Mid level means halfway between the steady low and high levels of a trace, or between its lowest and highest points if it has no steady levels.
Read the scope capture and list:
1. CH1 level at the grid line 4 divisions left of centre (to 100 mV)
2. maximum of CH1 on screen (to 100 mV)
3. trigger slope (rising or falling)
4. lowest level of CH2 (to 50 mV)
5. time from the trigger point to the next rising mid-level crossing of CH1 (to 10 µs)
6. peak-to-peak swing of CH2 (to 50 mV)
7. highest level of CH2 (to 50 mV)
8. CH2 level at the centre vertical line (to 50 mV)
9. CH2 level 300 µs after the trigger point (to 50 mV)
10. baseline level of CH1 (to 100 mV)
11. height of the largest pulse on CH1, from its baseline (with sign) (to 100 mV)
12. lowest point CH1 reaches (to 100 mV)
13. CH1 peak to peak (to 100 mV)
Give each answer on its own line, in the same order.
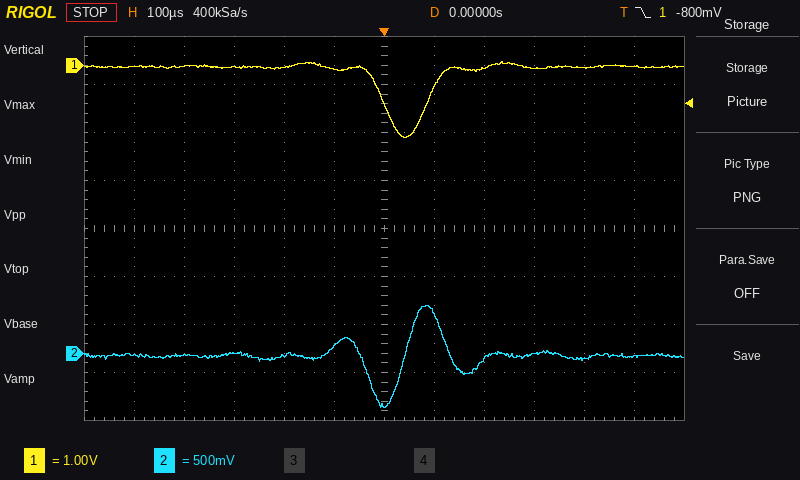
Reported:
0.0 V
100 mV
falling
-550 mV
90 µs
1.05 V
500 mV
-550 mV
0 mV
0.0 V
-1.5 V
-1.5 V
1.6 V
